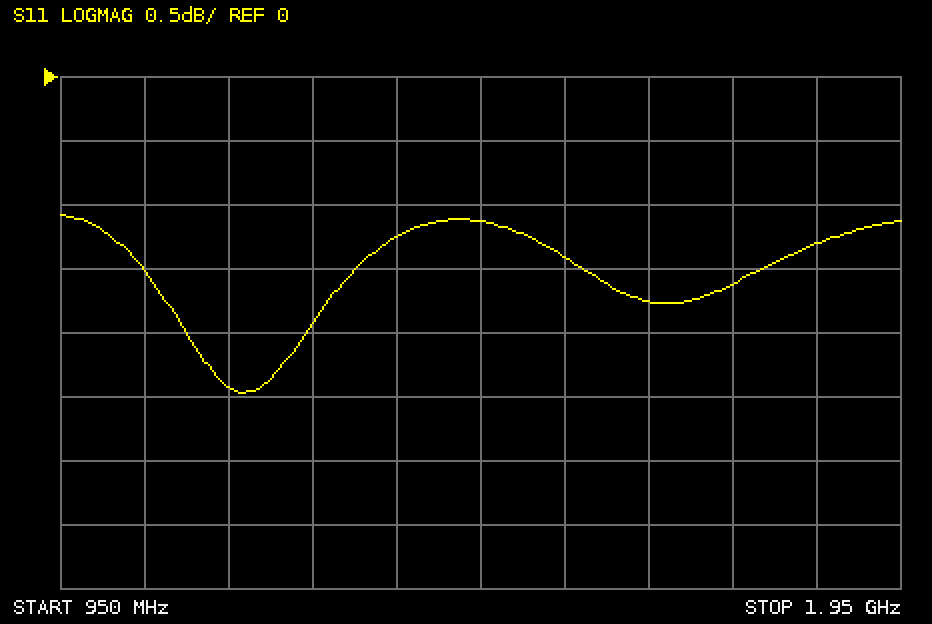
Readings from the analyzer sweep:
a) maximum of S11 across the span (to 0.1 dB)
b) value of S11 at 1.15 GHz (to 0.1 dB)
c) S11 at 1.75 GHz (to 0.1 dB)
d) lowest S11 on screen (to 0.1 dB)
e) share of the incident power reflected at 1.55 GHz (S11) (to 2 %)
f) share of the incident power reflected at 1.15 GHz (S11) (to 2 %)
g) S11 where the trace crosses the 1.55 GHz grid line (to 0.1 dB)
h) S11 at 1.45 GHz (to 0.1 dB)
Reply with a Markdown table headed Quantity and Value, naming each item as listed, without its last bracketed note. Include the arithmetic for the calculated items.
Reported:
| Quantity | Value |
|---|---|
| maximum of S11 across the span | -1.1 dB |
| value of S11 at 1.15 GHz | -2.4 dB |
| S11 at 1.75 GHz | -1.6 dB |
| lowest S11 on screen | -2.5 dB |
| share of the incident power reflected at 1.55 GHz (S11) | 10^(-1.4/10) ≈ 72 % |
| share of the incident power reflected at 1.15 GHz (S11) | 10^(-2.4/10) ≈ 58 % |
| S11 where the trace crosses the 1.55 GHz grid line | -1.4 dB |
| S11 at 1.45 GHz | -1.1 dB |
